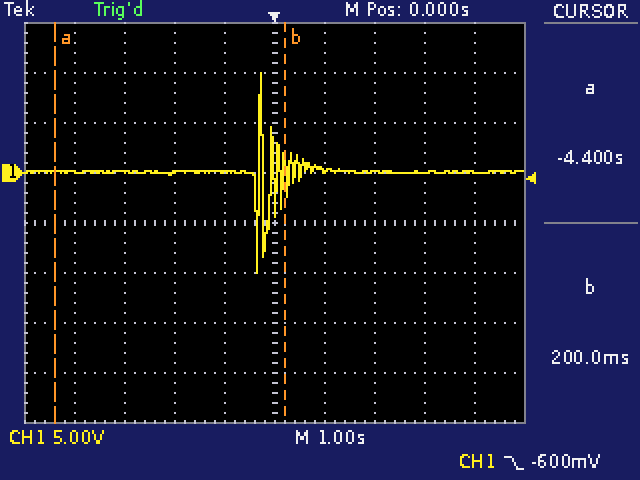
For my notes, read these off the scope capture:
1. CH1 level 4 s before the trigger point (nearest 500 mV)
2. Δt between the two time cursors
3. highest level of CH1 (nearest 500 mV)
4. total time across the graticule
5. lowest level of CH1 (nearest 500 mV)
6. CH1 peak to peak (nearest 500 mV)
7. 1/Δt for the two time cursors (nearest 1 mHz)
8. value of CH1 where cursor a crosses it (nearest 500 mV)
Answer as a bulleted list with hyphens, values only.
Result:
- 0.0 V
- 4.6 s
- 10.0 V
- 10 s
- -10.0 V
- 20.0 V
- 217 mHz
- 0.0 V
